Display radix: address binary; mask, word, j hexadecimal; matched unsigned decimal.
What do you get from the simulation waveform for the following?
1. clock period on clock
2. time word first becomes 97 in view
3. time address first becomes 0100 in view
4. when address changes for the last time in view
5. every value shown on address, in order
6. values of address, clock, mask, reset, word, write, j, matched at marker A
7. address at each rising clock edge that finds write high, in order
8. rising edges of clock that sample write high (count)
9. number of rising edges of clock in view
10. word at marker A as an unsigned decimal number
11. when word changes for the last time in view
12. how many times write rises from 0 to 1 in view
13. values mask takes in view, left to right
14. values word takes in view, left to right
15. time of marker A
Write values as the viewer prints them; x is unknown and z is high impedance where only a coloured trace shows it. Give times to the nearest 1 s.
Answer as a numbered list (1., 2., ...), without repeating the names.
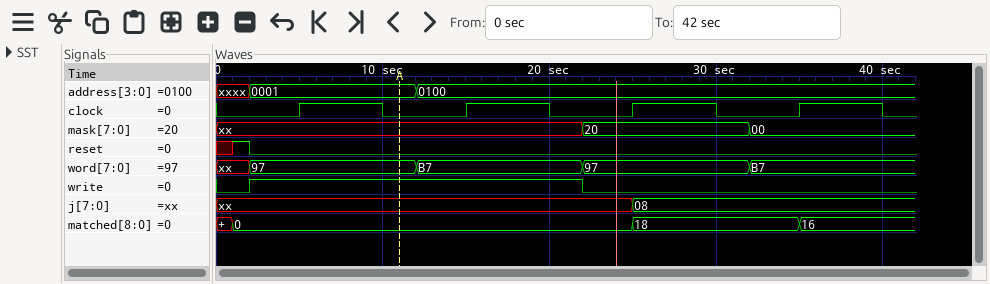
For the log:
1. 10 s
2. 2 s
3. 12 s
4. 12 s
5. xxxx, 0001, 0100
6. address=0001, clock=0, mask=xx, reset=0, word=97, write=1, j=xx, matched=0
7. 0001, 0100
8. 2
9. 4
10. 151
11. 32 s
12. 1
13. xx, 20, 00
14. xx, 97, B7, 97, B7
15. 11 s
